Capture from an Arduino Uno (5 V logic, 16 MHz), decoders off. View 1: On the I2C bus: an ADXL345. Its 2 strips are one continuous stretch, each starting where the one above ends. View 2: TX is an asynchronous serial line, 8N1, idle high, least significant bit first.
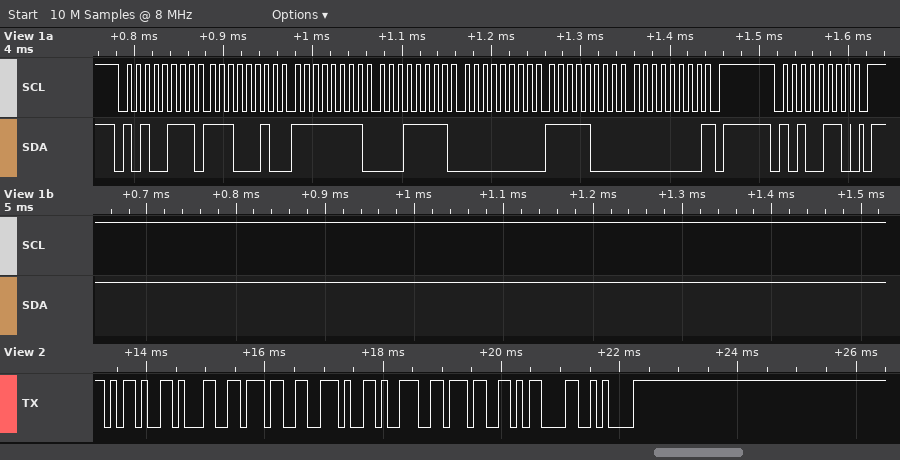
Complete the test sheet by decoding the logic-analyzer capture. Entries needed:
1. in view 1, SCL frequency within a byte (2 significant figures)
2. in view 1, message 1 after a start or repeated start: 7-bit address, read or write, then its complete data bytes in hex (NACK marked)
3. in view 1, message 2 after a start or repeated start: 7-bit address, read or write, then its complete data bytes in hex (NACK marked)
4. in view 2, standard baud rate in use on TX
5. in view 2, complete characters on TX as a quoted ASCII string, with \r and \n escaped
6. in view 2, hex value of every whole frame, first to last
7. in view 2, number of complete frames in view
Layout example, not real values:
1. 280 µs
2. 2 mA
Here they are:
1. 100 kHz
2. 0x53 read: E2 FF 1F 00 F8 00 NACK
3. 0x53 write
4. 9600 baud
5. "-17.97\r\n"
6. 2D 31 37 2E 39 37 0D 0A
7. 8
